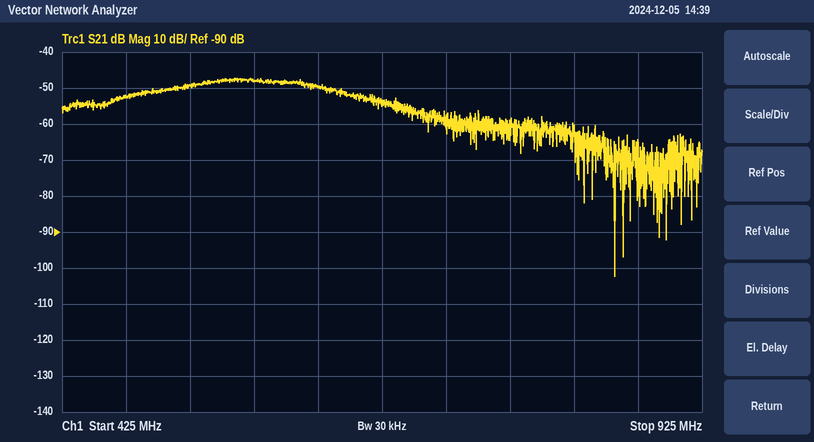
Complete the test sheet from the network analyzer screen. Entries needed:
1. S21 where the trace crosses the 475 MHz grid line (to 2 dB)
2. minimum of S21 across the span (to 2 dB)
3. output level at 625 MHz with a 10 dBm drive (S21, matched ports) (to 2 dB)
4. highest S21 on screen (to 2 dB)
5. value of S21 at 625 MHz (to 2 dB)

-52 dB
-102 dB
-40 dBm
-48 dB
-50 dB
